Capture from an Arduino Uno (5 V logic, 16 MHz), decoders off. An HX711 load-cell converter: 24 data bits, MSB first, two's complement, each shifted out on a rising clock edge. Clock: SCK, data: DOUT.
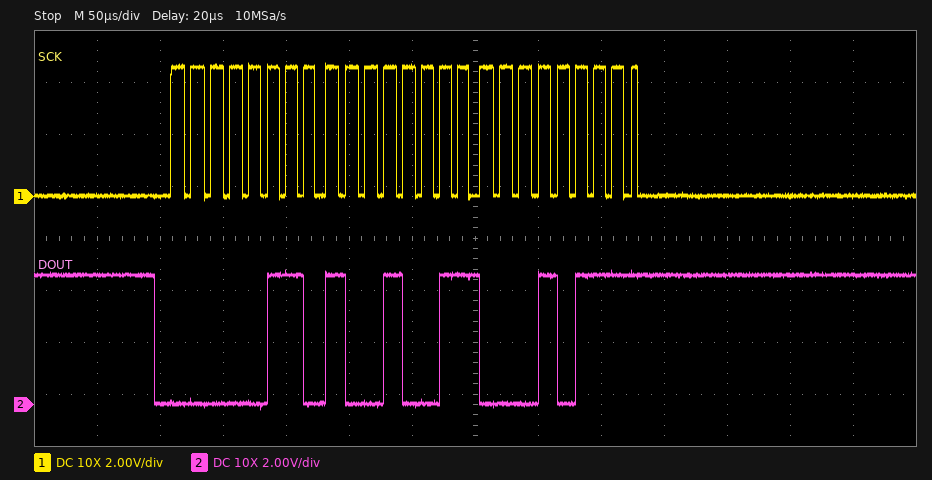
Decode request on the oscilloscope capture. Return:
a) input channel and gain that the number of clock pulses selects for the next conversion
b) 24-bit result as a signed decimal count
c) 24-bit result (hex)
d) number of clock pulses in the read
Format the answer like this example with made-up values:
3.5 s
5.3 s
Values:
channel A, gain 128
430871
0x069317
25
